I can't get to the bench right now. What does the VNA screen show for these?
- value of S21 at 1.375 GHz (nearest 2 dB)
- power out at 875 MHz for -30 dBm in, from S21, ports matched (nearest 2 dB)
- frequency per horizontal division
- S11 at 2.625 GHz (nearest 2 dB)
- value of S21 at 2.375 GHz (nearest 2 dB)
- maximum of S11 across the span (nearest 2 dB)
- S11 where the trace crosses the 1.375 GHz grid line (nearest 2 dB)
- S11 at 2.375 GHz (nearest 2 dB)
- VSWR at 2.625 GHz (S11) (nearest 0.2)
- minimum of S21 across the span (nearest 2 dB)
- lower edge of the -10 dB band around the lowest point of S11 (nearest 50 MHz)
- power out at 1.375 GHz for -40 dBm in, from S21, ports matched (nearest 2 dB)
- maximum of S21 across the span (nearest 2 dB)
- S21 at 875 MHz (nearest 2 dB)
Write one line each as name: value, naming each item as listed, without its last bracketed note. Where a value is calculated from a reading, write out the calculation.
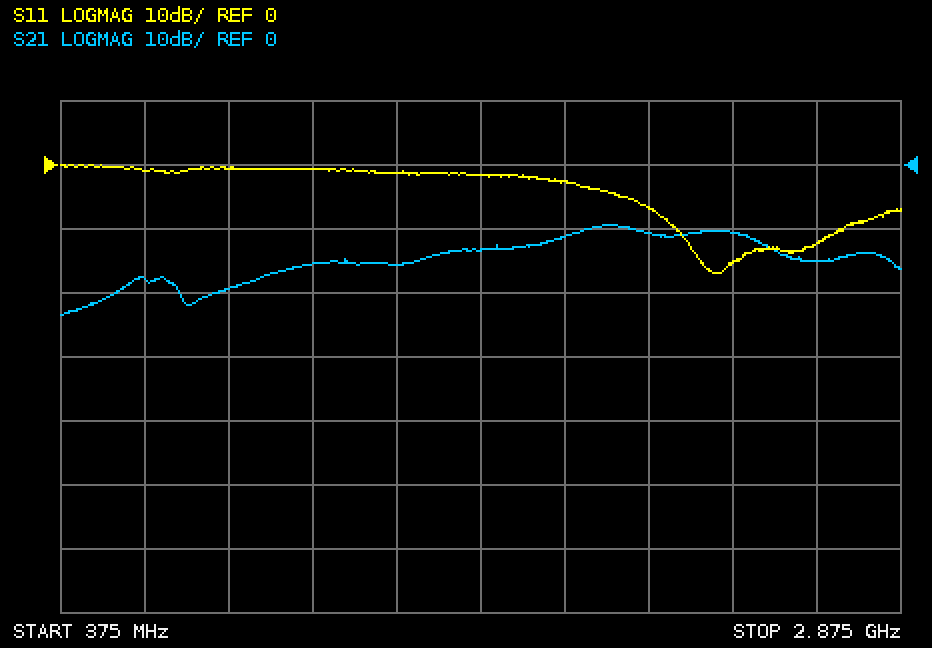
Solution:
value of S21 at 1.375 GHz: -16 dB
power out at 875 MHz for -30 dBm in, from S21, ports matched: -30 dBm + (-20 dB) = -50 dBm
frequency per horizontal division: 250 MHz
S11 at 2.625 GHz: -12 dB
value of S21 at 2.375 GHz: -10 dB
maximum of S11 across the span: 0 dB
S11 where the trace crosses the 1.375 GHz grid line: -2 dB
S11 at 2.375 GHz: -16 dB
VSWR at 2.625 GHz (S11): |Γ| = 10^(-12/20) = 0.2512; VSWR = (1 + 0.2512)/(1 − 0.2512) ≈ 1.67, so 1.6 to the nearest 0.2
minimum of S21 across the span: -24 dB
lower edge of the -10 dB band around the lowest point of S11: 2.20 GHz
power out at 1.375 GHz for -40 dBm in, from S21, ports matched: -40 dBm + (-16 dB) = -56 dBm
maximum of S21 across the span: -10 dB
S21 at 875 MHz: -20 dB
